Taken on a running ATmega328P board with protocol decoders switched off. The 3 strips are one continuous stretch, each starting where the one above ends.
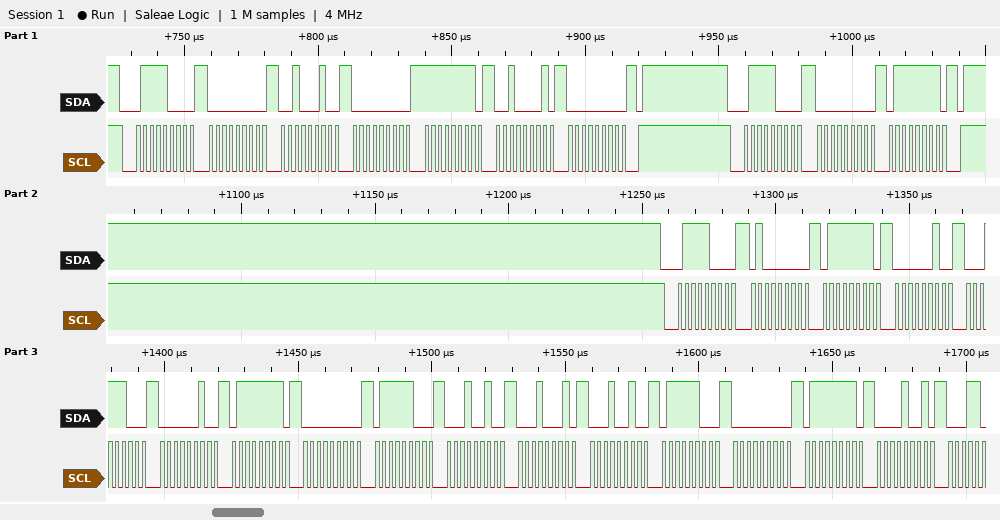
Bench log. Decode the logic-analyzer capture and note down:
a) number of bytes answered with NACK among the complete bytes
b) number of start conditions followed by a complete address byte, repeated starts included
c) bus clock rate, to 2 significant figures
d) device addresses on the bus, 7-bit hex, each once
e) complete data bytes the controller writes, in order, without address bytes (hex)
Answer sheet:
0
3
400 kHz
0x3C
00 22 00 FF 21 00 00 7F 40 7F 02 1C 02 7F 00 7C 12 11 12 7C 00 7F 09
